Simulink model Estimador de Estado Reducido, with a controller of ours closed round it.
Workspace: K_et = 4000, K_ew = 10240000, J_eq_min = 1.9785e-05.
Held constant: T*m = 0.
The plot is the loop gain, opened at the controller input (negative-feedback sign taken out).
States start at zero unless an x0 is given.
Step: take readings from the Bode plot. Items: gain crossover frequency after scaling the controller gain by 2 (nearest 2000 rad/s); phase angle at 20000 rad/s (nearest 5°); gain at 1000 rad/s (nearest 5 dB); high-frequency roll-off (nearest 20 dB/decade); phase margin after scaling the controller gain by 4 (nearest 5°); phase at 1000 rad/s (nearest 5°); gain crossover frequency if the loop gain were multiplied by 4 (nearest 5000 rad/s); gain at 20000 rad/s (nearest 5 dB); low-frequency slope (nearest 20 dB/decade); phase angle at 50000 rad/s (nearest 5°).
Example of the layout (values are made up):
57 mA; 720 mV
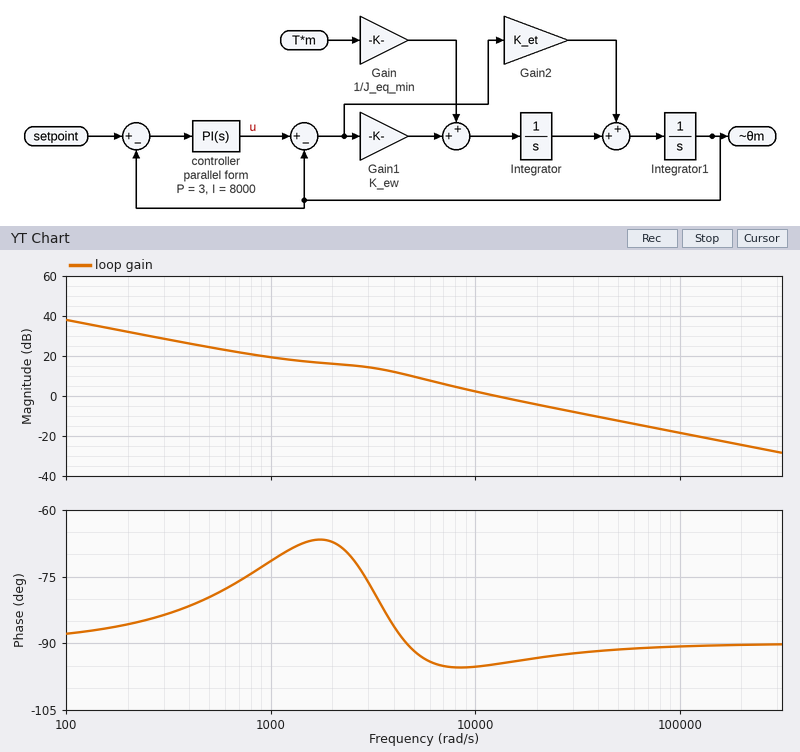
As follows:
24000 rad/s; -95°; 20 dB; -20 dB/decade; 90°; -70°; 50000 rad/s; -5 dB; -20 dB/decade; -90°
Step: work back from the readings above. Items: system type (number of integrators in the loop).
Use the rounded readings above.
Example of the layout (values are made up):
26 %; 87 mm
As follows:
1
